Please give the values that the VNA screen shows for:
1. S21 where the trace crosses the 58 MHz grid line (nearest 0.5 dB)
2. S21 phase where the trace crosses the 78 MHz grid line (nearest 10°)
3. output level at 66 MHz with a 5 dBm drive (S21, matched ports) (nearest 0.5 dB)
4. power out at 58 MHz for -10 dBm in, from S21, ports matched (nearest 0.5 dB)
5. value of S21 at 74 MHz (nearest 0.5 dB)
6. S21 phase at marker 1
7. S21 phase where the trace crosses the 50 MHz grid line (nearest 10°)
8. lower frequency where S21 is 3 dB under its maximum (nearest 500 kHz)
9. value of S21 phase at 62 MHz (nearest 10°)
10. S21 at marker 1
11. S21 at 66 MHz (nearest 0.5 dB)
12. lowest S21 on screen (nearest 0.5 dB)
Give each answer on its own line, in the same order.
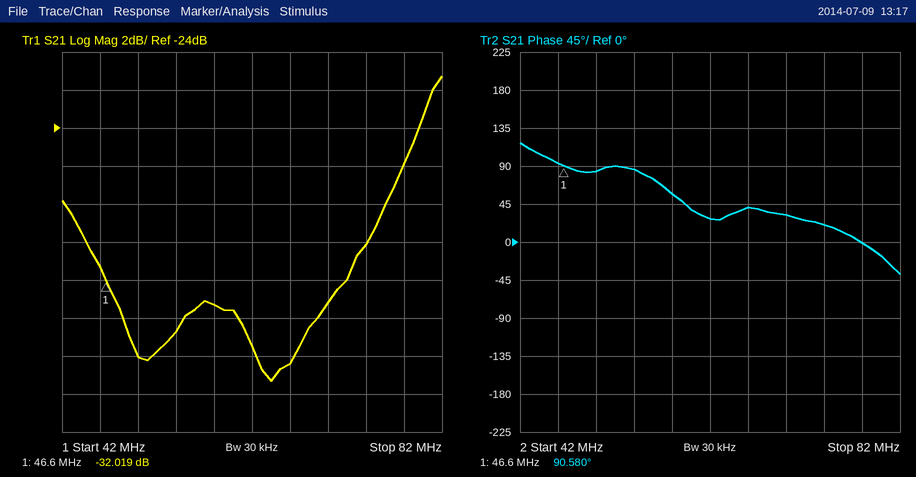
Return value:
-33.5 dB
0°
-31.5 dBm
-43.5 dBm
-30.0 dB
90.580°
80°
79.5 MHz
30°
-32.019 dB
-36.5 dB
-37.5 dB
